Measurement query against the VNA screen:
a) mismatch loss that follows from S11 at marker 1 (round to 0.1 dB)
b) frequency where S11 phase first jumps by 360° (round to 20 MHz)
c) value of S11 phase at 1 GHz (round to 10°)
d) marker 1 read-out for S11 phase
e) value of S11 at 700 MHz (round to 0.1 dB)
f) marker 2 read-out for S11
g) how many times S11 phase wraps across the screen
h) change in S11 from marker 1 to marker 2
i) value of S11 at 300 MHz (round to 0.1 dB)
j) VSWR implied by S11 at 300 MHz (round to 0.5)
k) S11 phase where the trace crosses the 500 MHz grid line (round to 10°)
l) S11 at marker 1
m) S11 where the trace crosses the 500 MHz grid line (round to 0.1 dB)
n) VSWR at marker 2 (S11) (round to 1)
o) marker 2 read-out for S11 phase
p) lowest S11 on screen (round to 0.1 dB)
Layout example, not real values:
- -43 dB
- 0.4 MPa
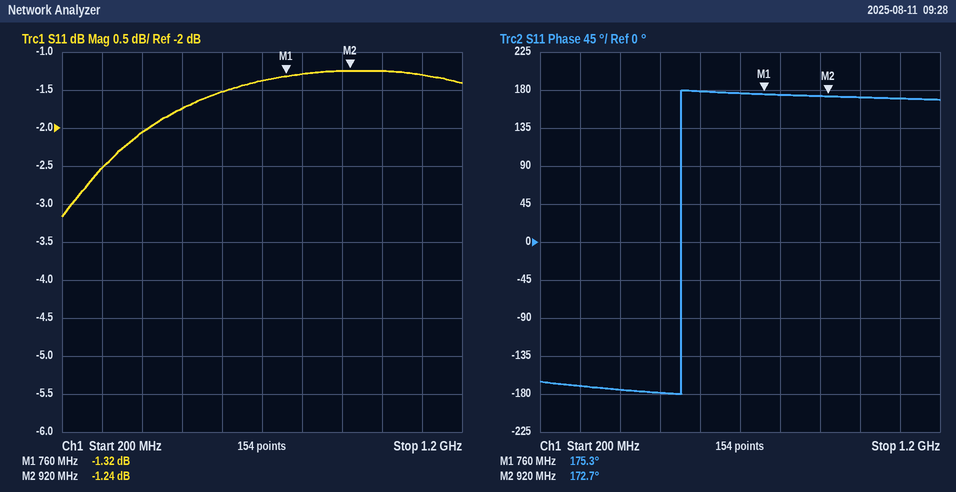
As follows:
- 5.8 dB
- 560 MHz
- 170°
- 175.3°
- -1.4 dB
- -1.24 dB
- 1
- 0.08 dB
- -2.5 dB
- 7.0
- -180°
- -1.32 dB
- -1.7 dB
- 14
- 172.7°
- -3.2 dB
